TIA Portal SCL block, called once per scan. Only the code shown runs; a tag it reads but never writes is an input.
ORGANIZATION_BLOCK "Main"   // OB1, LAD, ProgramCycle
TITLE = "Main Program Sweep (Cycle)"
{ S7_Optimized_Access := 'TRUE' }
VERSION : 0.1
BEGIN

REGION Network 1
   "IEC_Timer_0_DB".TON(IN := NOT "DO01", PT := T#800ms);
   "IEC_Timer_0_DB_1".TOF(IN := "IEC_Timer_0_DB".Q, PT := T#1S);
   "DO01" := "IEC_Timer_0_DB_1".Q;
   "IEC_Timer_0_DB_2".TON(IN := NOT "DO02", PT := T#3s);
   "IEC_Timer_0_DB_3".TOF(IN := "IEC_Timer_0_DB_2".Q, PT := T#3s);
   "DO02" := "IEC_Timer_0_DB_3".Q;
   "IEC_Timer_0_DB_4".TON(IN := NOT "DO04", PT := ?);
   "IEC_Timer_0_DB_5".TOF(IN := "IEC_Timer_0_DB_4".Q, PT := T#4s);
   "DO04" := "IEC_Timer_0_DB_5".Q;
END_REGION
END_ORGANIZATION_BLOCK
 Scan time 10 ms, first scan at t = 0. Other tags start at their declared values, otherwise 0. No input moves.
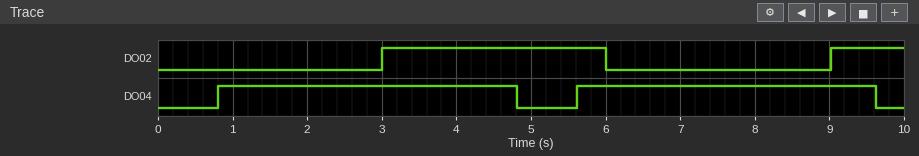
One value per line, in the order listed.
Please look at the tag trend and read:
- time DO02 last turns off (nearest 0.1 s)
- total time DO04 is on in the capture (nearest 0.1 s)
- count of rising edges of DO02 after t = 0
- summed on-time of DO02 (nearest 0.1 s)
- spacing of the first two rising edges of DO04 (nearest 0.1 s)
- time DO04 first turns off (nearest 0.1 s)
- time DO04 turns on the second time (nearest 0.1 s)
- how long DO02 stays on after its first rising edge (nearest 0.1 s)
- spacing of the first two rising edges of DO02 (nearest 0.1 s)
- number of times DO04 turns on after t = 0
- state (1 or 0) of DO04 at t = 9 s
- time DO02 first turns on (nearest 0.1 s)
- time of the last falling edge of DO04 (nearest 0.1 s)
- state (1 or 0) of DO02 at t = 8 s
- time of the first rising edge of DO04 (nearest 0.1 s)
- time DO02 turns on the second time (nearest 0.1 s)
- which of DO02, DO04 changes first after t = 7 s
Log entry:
6.0 s
8.0 s
2
4.0 s
4.8 s
4.8 s
5.6 s
3.0 s
6.0 s
2
1
3.0 s
9.6 s
0
0.8 s
9.0 s
DO02
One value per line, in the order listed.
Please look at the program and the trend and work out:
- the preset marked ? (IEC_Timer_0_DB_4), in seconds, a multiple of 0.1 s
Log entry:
0.8 s
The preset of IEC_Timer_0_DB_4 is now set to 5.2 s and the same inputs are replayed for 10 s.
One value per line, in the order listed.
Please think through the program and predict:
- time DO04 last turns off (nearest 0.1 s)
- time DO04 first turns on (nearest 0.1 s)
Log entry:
9.2 s
5.2 s
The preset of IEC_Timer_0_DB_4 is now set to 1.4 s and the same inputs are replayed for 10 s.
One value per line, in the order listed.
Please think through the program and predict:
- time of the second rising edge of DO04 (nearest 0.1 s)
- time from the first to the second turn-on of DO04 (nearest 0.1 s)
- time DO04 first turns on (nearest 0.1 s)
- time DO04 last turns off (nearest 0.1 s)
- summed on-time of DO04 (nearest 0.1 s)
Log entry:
6.8 s
5.4 s
1.4 s
5.4 s
7.2 s
